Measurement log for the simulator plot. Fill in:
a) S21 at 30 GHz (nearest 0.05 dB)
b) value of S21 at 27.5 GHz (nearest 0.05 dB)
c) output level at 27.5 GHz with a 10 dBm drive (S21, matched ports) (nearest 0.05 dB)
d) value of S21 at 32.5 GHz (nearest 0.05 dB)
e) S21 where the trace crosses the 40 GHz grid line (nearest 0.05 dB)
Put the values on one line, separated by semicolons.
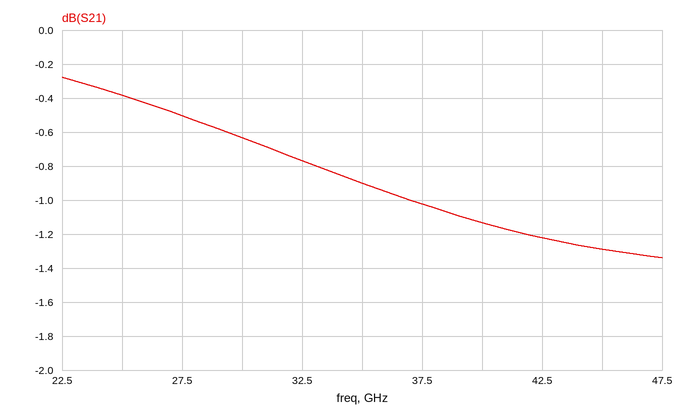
-0.65 dB; -0.50 dB; 9.50 dBm; -0.75 dB; -1.15 dB
